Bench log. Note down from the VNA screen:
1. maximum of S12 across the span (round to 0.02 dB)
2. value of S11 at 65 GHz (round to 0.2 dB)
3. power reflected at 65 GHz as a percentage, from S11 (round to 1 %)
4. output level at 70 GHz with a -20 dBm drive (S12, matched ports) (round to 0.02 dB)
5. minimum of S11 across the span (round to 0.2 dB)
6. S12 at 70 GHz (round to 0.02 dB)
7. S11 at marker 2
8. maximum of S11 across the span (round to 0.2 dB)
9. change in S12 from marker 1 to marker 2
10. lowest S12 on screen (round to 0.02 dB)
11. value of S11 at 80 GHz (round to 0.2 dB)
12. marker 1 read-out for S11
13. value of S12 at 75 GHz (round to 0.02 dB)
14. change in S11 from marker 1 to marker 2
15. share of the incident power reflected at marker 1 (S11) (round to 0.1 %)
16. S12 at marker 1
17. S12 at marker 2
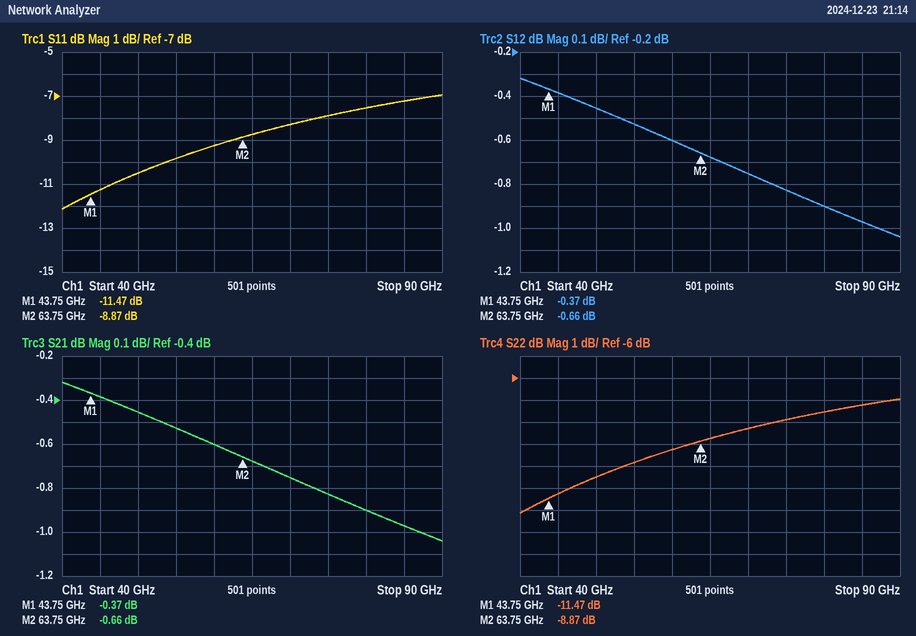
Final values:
-0.32 dB
-8.8 dB
13 %
-20.76 dBm
-12.2 dB
-0.76 dB
-8.87 dB
-7.0 dB
-0.29 dB
-1.04 dB
-7.6 dB
-11.47 dB
-0.82 dB
2.60 dB
7.1 %
-0.37 dB
-0.66 dB
